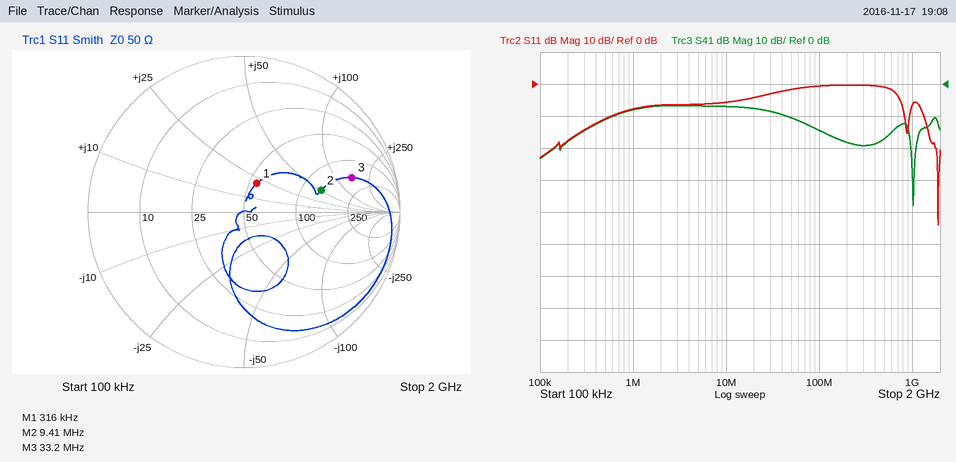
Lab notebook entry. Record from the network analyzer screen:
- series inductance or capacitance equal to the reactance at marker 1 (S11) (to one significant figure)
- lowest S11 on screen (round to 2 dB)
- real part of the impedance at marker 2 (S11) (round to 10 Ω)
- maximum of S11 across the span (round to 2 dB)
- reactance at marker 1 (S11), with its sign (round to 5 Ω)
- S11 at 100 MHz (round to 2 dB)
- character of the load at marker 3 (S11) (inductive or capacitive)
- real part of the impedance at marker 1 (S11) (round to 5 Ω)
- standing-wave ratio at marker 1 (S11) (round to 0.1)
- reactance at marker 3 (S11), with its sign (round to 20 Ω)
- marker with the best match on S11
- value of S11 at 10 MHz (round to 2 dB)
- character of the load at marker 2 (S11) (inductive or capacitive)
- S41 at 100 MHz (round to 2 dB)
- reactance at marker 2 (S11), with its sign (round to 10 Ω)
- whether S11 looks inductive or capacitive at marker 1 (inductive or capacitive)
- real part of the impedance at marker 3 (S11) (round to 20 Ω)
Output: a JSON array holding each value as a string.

["10 µH", "-44 dB", "130 Ω", "0 dB", "+20 Ω", "0 dB", "inductive", "55 Ω", "1.5", "+160 Ω", "marker 1", "-6 dB", "inductive", "-14 dB", "+50 Ω", "inductive", "160 Ω"]
